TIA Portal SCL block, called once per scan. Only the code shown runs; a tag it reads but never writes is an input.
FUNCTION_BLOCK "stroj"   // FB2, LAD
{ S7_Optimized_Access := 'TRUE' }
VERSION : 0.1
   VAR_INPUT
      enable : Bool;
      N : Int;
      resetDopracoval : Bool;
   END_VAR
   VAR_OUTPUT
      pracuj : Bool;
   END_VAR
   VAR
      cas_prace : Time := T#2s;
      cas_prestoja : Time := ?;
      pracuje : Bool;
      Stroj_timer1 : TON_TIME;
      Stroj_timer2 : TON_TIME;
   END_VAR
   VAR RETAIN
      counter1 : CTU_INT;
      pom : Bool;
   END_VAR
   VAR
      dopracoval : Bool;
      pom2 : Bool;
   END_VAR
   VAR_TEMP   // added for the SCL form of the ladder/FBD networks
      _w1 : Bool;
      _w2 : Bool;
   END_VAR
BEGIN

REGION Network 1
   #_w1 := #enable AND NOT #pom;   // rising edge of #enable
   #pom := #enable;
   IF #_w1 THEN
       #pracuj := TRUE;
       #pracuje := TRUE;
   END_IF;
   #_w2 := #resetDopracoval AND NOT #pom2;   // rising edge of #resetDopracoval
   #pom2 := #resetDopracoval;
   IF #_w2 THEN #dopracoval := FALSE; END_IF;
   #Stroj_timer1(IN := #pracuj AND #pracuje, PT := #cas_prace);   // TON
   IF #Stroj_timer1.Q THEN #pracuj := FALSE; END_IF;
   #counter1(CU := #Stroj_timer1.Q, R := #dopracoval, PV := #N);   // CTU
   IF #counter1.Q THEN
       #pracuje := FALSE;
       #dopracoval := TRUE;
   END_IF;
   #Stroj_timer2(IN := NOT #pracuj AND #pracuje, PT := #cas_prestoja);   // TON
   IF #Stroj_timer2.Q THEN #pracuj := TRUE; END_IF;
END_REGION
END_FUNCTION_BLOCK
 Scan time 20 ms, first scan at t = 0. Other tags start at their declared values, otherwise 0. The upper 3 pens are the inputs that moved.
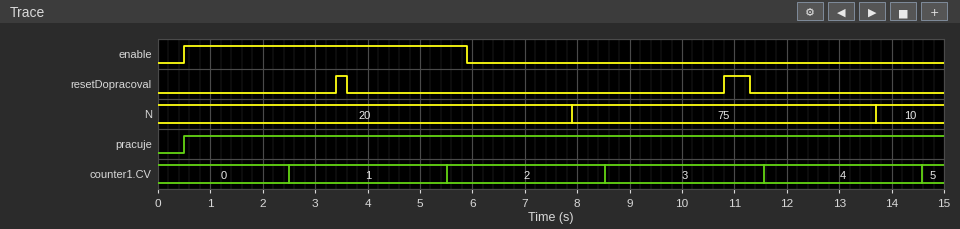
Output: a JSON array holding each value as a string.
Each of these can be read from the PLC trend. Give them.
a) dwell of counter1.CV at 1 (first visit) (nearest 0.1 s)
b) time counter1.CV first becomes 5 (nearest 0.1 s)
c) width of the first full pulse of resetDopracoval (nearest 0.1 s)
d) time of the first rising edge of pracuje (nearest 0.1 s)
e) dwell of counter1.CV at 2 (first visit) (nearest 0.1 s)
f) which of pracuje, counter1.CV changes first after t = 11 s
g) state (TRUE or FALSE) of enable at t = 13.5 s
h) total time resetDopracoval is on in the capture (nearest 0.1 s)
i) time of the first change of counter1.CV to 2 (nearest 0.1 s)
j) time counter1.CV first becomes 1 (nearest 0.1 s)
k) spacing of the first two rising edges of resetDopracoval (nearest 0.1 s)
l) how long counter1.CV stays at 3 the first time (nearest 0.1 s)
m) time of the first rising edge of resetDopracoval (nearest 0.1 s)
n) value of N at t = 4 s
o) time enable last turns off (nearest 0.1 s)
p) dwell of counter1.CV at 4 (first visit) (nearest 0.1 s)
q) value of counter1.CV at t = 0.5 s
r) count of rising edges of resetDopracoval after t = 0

["3.0 s", "14.6 s", "0.2 s", "0.5 s", "3.0 s", "counter1.CV", "FALSE", "0.7 s", "5.5 s", "2.5 s", "7.4 s", "3.0 s", "3.4 s", "20", "5.9 s", "3.0 s", "0", "2"]
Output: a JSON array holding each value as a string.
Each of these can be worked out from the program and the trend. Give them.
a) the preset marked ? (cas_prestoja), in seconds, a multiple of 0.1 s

["1.0 s"]
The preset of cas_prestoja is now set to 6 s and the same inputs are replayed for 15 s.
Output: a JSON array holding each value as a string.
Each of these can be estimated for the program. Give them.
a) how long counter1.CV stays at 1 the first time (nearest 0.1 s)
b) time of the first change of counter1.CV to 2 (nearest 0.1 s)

["8.0 s", "10.5 s"]
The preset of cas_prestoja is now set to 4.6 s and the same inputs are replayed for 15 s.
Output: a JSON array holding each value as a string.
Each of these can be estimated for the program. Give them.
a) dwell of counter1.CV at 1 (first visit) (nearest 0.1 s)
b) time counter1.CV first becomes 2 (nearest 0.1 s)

["6.6 s", "9.1 s"]
